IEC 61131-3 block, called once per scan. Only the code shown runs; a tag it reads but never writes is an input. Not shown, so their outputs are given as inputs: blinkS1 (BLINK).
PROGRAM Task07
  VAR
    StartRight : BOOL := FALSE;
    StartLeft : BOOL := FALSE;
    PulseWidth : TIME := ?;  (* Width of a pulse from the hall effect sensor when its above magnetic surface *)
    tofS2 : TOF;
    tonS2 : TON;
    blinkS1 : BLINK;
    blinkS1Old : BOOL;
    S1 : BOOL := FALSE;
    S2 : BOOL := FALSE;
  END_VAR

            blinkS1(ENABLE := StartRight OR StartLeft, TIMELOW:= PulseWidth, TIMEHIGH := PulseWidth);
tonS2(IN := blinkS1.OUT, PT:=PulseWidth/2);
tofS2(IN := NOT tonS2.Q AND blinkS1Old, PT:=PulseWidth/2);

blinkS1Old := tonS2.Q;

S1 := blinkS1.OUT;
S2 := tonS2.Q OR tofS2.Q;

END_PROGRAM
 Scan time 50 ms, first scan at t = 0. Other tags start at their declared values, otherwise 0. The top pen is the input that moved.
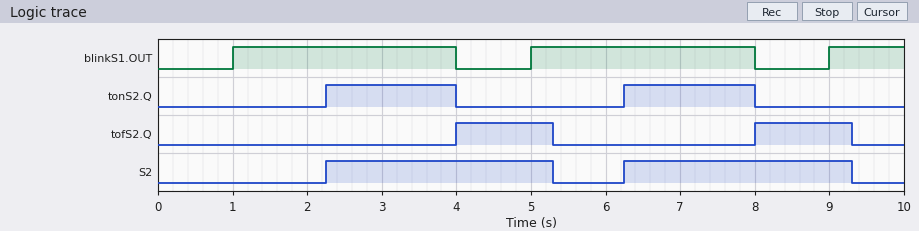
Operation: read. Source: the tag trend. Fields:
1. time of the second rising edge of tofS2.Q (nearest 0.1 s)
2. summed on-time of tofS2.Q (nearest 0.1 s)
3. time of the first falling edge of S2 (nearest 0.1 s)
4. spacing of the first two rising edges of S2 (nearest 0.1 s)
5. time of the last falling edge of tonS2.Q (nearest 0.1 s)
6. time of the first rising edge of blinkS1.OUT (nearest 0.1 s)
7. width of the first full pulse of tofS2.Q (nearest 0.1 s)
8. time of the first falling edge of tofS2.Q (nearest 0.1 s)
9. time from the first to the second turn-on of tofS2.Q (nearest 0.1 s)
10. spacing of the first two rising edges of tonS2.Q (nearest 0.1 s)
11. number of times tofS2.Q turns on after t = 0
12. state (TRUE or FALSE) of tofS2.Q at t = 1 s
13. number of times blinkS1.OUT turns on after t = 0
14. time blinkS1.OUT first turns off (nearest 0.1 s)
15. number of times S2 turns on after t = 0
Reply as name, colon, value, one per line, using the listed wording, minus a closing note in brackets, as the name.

time of the second rising edge of tofS2.Q: 8.0 s
summed on-time of tofS2.Q: 2.6 s
time of the first falling edge of S2: 5.3 s
spacing of the first two rising edges of S2: 4.0 s
time of the last falling edge of tonS2.Q: 8.0 s
time of the first rising edge of blinkS1.OUT: 1.0 s
width of the first full pulse of tofS2.Q: 1.3 s
time of the first falling edge of tofS2.Q: 5.3 s
time from the first to the second turn-on of tofS2.Q: 4.0 s
spacing of the first two rising edges of tonS2.Q: 4.0 s
number of times tofS2.Q turns on after t = 0: 2
state (TRUE or FALSE) of tofS2.Q at t = 1 s: FALSE
number of times blinkS1.OUT turns on after t = 0: 3
time blinkS1.OUT first turns off: 4.0 s
number of times S2 turns on after t = 0: 2
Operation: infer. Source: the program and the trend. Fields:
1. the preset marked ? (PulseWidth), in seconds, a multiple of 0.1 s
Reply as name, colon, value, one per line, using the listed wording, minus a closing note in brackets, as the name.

the preset marked ? (PulseWidth), in seconds, a multiple of 0.1 s: 2.5 s
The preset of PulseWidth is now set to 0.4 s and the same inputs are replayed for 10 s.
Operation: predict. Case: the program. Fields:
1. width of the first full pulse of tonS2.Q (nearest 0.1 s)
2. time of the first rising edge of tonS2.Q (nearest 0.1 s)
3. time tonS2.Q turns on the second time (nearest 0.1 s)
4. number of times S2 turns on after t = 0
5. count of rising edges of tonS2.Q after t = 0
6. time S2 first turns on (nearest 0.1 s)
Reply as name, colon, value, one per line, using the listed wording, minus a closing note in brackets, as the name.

width of the first full pulse of tonS2.Q: 2.8 s
time of the first rising edge of tonS2.Q: 1.2 s
time tonS2.Q turns on the second time: 5.2 s
number of times S2 turns on after t = 0: 3
count of rising edges of tonS2.Q after t = 0: 3
time S2 first turns on: 1.2 s
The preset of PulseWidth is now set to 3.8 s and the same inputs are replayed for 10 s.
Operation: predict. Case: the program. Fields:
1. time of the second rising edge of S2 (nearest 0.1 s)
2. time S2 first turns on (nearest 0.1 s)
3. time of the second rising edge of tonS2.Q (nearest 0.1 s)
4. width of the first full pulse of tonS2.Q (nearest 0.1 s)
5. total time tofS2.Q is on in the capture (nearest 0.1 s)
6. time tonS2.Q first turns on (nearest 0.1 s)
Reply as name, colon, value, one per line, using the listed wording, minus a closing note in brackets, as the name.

time of the second rising edge of S2: 6.9 s
time S2 first turns on: 2.9 s
time of the second rising edge of tonS2.Q: 6.9 s
width of the first full pulse of tonS2.Q: 1.1 s
total time tofS2.Q is on in the capture: 3.9 s
time tonS2.Q first turns on: 2.9 s
